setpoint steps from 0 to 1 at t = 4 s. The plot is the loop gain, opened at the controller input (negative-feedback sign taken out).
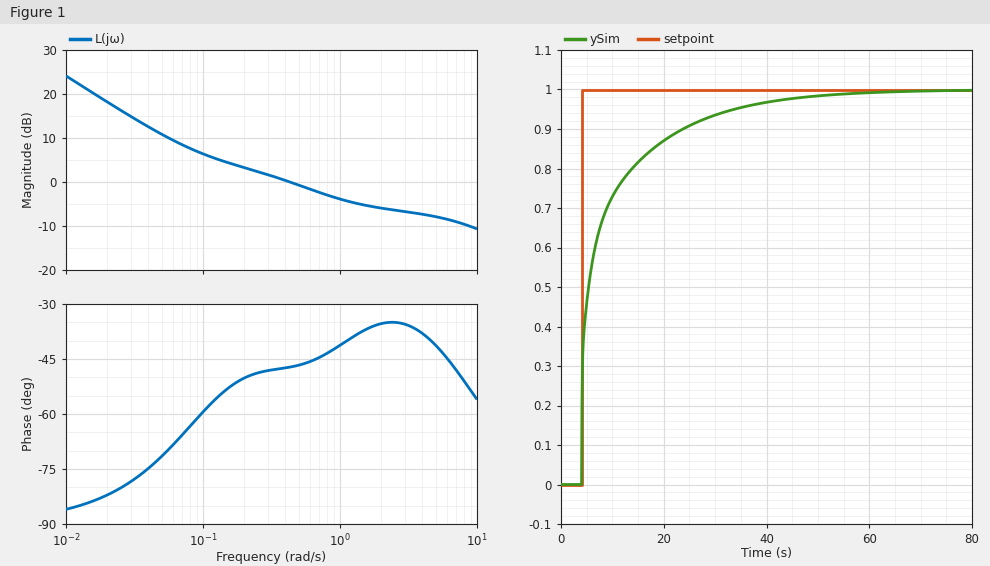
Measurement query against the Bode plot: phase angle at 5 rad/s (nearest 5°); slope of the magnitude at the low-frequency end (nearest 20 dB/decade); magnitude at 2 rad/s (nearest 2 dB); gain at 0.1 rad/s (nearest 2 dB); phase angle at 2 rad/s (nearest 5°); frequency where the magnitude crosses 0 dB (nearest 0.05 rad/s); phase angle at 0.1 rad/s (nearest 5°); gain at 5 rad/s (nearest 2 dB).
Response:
-40°
-20 dB/decade
-6 dB
6 dB
-35°
0.45 rad/s
-60°
-8 dB
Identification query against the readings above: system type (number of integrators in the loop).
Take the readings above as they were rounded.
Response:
1
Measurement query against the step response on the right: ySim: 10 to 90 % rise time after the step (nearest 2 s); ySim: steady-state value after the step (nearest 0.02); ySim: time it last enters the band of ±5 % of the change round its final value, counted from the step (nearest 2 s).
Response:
20 s
1.00
30 s
